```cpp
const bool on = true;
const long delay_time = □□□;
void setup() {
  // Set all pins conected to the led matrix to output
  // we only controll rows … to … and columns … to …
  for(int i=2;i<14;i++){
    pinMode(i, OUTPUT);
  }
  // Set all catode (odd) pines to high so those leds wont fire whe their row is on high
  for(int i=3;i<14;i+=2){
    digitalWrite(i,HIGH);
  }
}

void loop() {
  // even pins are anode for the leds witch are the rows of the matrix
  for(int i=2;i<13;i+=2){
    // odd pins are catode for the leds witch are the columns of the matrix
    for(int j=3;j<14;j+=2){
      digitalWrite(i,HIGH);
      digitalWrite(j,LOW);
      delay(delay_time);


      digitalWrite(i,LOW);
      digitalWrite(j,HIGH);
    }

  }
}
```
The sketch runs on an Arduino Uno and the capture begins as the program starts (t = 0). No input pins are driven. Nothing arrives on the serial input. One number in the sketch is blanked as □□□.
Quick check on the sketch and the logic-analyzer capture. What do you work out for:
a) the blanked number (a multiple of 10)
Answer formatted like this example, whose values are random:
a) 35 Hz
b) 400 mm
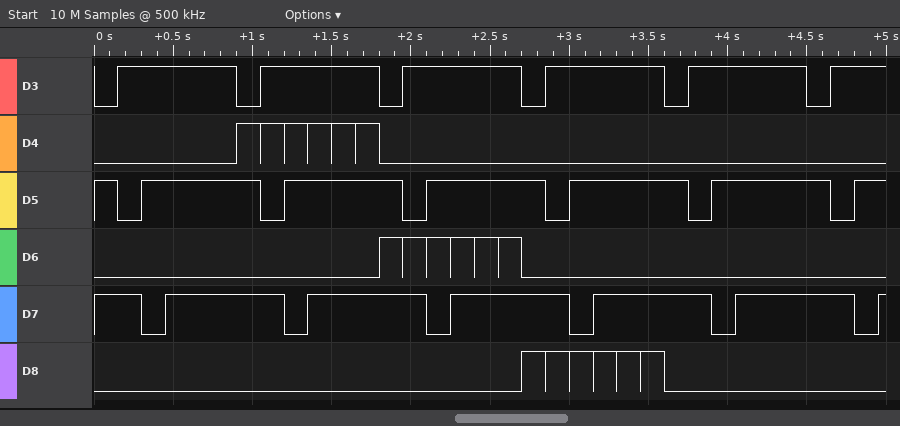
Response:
a) 150
